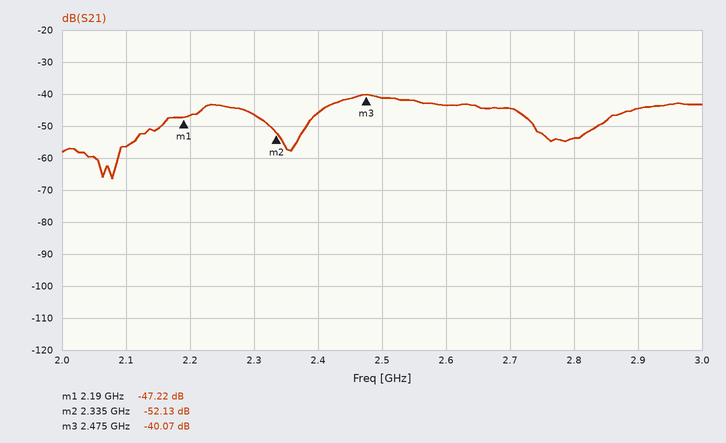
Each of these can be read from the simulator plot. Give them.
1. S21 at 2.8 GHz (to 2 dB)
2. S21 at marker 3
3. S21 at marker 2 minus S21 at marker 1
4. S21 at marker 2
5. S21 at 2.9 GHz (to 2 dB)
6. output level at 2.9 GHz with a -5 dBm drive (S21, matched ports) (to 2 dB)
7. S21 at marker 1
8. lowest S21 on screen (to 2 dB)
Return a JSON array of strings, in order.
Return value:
["-54 dB", "-40.07 dB", "-4.91 dB", "-52.13 dB", "-44 dB", "-50 dBm", "-47.22 dB", "-66 dB"]
